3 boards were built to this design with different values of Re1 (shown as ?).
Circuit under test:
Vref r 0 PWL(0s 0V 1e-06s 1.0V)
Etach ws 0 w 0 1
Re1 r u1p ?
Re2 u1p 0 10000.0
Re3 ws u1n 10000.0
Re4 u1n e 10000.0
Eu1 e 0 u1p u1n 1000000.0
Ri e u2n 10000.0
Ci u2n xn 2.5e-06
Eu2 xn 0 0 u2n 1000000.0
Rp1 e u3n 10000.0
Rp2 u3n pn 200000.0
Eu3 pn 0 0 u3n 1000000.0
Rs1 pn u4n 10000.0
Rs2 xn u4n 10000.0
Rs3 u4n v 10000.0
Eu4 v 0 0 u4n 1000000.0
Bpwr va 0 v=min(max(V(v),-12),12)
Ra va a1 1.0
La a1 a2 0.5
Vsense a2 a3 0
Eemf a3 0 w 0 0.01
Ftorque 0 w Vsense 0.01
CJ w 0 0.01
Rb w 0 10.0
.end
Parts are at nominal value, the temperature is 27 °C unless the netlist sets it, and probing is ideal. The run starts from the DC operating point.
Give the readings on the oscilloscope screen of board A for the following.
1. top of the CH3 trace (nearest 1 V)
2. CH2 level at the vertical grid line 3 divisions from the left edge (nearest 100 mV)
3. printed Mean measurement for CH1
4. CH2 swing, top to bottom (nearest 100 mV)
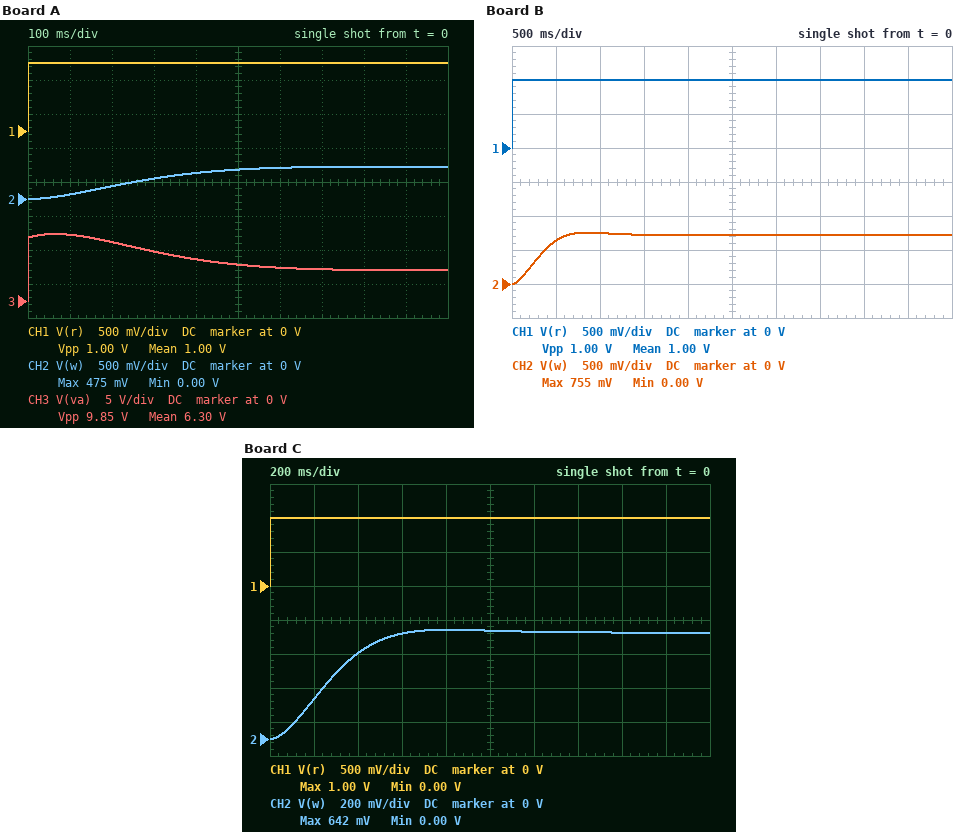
10 V
300 mV
1.00 V
500 mV
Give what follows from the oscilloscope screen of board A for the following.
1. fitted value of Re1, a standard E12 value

33 kΩ
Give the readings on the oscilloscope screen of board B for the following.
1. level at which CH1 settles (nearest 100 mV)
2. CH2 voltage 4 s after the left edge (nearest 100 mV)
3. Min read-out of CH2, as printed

1.0 V
700 mV
0.00 V
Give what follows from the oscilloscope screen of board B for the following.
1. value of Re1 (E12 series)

18 kΩ
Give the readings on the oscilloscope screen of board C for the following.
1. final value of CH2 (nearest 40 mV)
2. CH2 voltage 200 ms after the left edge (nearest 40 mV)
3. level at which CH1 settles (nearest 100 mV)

640 mV
240 mV
1.0 V
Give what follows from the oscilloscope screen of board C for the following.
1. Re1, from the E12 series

22 kΩ
